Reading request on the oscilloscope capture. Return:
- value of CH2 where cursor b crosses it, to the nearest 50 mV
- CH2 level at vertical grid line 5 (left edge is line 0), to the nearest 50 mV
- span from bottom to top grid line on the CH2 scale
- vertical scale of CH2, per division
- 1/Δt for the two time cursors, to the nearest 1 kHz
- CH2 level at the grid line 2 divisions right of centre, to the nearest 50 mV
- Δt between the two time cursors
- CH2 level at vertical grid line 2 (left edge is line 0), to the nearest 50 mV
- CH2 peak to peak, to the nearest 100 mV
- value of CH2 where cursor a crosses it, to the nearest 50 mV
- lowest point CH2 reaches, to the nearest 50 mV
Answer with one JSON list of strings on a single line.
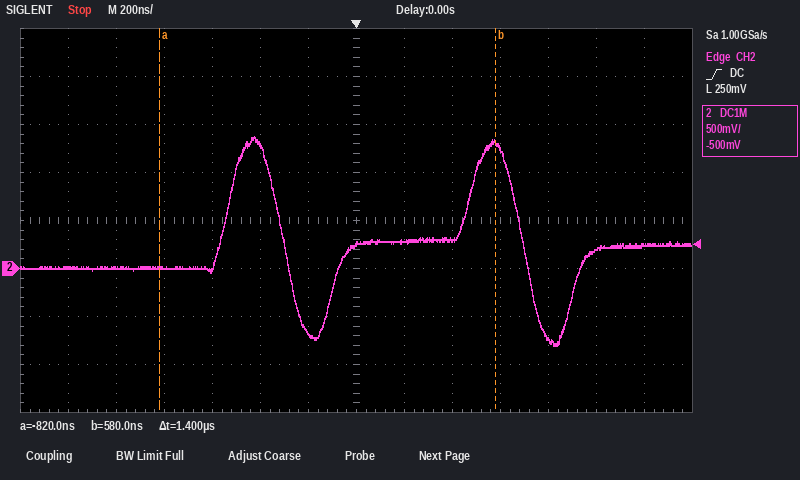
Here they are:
["1.30 V", "1.30 V", "4 V", "500 mV", "714 kHz", "300 mV", "1.4 µs", "0 mV", "2.20 V", "0 mV", "-800 mV"]
